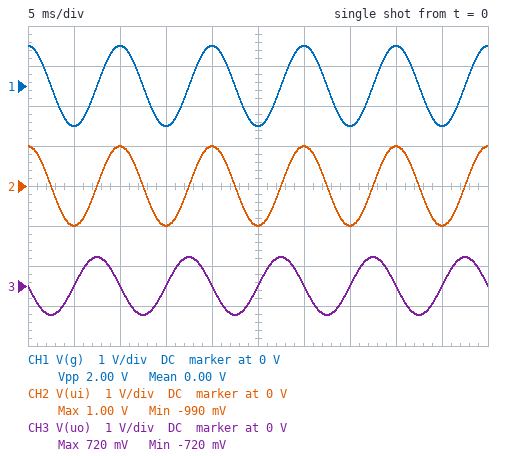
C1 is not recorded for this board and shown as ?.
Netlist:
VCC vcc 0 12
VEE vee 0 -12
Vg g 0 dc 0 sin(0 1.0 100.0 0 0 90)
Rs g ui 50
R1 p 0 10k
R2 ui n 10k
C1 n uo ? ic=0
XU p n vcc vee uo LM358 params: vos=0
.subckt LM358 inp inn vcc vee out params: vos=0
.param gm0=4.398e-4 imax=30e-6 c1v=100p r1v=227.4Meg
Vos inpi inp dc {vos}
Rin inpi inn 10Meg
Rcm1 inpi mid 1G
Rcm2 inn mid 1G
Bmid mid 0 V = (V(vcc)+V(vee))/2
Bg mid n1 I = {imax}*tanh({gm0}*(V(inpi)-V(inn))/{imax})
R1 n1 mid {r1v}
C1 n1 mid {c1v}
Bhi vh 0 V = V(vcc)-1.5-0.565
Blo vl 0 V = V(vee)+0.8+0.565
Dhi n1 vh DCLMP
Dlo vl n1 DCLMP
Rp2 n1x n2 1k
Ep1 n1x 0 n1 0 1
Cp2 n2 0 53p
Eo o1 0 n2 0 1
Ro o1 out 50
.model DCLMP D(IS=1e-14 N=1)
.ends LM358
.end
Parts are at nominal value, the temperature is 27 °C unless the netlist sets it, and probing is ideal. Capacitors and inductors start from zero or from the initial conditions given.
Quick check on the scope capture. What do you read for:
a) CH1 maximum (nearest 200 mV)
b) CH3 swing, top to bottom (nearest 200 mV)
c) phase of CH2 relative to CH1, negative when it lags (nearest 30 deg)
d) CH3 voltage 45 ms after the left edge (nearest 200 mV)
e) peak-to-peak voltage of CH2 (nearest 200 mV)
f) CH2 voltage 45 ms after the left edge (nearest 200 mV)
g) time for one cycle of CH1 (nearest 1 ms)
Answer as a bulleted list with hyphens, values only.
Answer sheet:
- 1.0 V
- 1.4 V
- 0 deg
- 0 V
- 2.0 V
- -1.0 V
- 10 ms
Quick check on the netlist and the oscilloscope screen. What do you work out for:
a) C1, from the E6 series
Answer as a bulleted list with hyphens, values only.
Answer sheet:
- 220 nF
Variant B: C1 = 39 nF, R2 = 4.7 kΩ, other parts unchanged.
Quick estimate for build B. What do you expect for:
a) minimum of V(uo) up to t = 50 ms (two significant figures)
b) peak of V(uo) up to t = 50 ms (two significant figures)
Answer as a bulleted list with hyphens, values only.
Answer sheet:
- -8.6 V
- 8.6 V
